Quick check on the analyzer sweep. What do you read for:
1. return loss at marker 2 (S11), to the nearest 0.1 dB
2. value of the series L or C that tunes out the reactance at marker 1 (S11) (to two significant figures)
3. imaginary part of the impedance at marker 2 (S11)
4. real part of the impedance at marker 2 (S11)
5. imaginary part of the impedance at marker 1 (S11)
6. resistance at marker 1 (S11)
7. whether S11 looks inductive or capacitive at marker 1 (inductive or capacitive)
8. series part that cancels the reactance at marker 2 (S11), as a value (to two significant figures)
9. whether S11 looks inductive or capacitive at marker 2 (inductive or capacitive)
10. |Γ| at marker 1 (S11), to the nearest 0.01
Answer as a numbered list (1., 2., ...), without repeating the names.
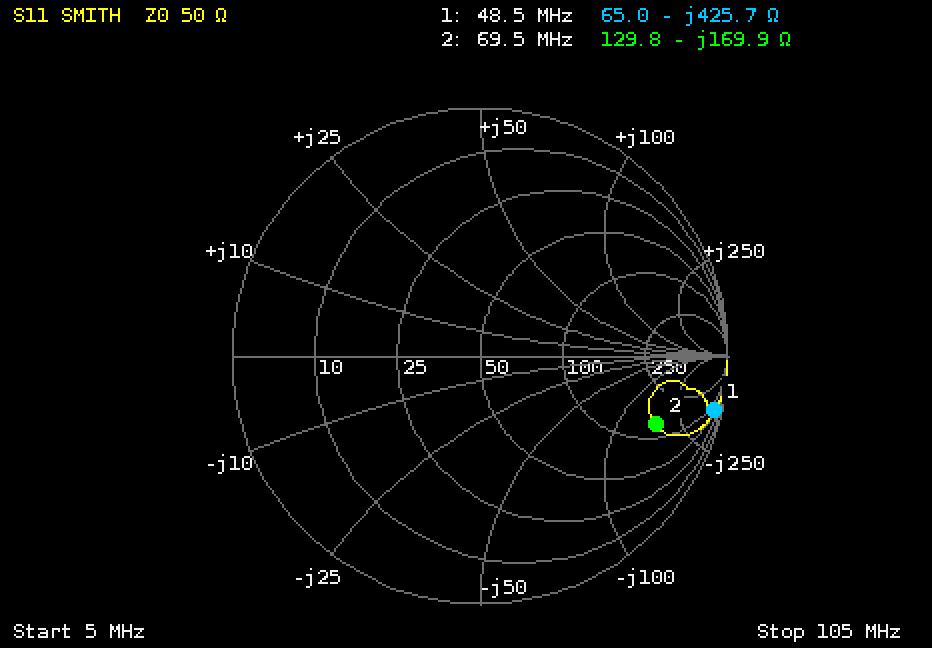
1. 2.4 dB
2. 1.4 µH
3. -169.9 Ω
4. 129.8 Ω
5. -425.7 Ω
6. 65.0 Ω
7. capacitive
8. 390 nH
9. capacitive
10. 0.97
